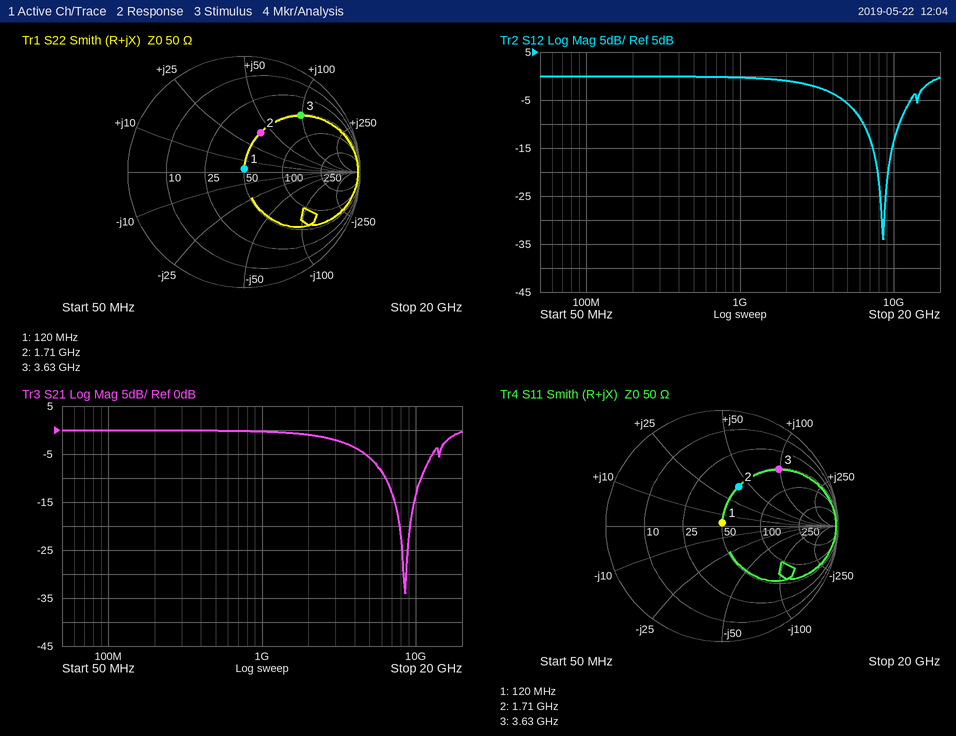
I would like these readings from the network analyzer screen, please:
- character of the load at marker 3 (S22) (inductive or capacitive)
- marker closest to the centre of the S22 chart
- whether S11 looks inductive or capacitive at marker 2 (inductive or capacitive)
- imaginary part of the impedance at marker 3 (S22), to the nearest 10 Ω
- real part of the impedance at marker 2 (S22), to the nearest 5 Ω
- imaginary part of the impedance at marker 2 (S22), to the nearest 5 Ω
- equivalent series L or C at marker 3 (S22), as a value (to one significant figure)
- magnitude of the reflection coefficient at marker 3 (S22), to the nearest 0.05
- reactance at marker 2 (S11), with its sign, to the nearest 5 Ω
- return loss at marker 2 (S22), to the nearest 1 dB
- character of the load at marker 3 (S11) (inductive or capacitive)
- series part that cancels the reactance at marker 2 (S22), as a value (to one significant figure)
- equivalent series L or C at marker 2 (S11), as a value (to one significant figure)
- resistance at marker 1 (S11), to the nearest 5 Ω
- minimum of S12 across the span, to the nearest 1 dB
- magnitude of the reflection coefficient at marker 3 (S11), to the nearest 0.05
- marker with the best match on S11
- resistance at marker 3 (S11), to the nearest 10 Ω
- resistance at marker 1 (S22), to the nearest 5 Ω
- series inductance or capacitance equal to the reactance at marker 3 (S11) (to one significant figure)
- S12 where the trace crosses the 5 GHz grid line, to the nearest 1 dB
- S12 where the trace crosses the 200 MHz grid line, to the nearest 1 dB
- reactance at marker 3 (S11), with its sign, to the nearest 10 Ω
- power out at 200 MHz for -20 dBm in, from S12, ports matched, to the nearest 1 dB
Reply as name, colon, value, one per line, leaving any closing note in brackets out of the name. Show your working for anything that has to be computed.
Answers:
character of the load at marker 3 (S22): inductive
marker closest to the centre of the S22 chart: marker 1
whether S11 looks inductive or capacitive at marker 2: inductive
imaginary part of the impedance at marker 3 (S22), to the nearest 10 Ω: +100 Ω
real part of the impedance at marker 2 (S22), to the nearest 5 Ω: 50 Ω
imaginary part of the impedance at marker 2 (S22), to the nearest 5 Ω: +40 Ω
equivalent series L or C at marker 3 (S22), as a value: L = 100 Ω/(2π × 3.63 GHz) ≈ 4 nH
magnitude of the reflection coefficient at marker 3 (S22), to the nearest 0.05: 0.70
reactance at marker 2 (S11), with its sign, to the nearest 5 Ω: +40 Ω
return loss at marker 2 (S22), to the nearest 1 dB: 9 dB
character of the load at marker 3 (S11): inductive
series part that cancels the reactance at marker 2 (S22), as a value: C = 1/(2π × 1.71 GHz × 40 Ω) ≈ 2 pF
equivalent series L or C at marker 2 (S11), as a value: L = 40 Ω/(2π × 1.71 GHz) ≈ 4 nH
resistance at marker 1 (S11), to the nearest 5 Ω: 50 Ω
minimum of S12 across the span, to the nearest 1 dB: -34 dB
magnitude of the reflection coefficient at marker 3 (S11), to the nearest 0.05: 0.70
marker with the best match on S11: marker 1
resistance at marker 3 (S11), to the nearest 10 Ω: 50 Ω
resistance at marker 1 (S22), to the nearest 5 Ω: 50 Ω
series inductance or capacitance equal to the reactance at marker 3 (S11): L = 100 Ω/(2π × 3.63 GHz) ≈ 4 nH
S12 where the trace crosses the 5 GHz grid line, to the nearest 1 dB: -6 dB
S12 where the trace crosses the 200 MHz grid line, to the nearest 1 dB: 0 dB
reactance at marker 3 (S11), with its sign, to the nearest 10 Ω: +100 Ω
power out at 200 MHz for -20 dBm in, from S12, ports matched, to the nearest 1 dB: -20 dBm + (0 dB) = -20 dBm
